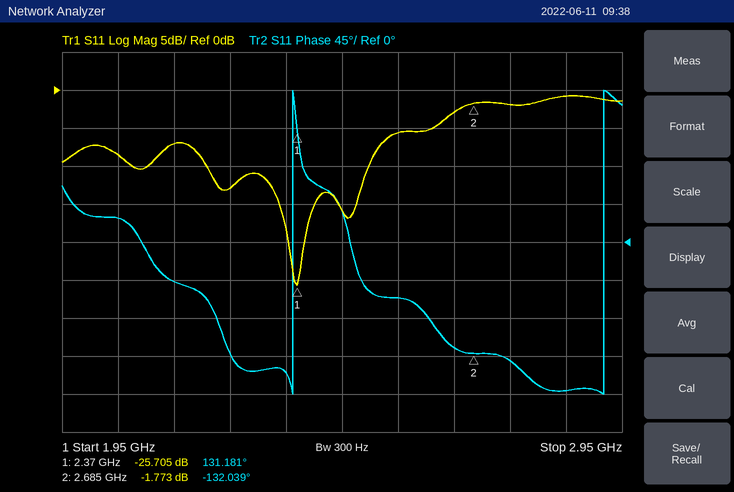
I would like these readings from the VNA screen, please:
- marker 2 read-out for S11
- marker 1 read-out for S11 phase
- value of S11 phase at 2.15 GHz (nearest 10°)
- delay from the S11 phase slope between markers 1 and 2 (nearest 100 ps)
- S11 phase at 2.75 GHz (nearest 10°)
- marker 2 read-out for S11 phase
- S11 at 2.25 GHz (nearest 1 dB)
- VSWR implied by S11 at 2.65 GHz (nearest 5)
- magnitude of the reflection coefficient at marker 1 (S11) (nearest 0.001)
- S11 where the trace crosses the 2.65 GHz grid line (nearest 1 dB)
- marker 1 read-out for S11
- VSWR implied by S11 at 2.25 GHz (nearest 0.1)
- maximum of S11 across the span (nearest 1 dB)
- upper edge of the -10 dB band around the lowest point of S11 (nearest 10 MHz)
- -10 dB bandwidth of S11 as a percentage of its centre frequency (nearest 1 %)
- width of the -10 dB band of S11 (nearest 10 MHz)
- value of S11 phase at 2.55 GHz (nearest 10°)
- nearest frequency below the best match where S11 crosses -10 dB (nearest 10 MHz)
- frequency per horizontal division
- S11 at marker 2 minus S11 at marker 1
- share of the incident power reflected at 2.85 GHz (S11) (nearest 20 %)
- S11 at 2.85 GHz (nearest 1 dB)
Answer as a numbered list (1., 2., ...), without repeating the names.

1. -1.773 dB
2. 131.181°
3. -50°
4. 2.3 ns
5. -140°
6. -132.039°
7. -13 dB
8. 5
9. 0.052
10. -3 dB
11. -25.705 dB
12. 1.6
13. -1 dB
14. 2.50 GHz
15. 12 %
16. 290 MHz
17. -70°
18. 2.21 GHz
19. 100 MHz
20. 23.932 dB
21. 80 %
22. -1 dB
